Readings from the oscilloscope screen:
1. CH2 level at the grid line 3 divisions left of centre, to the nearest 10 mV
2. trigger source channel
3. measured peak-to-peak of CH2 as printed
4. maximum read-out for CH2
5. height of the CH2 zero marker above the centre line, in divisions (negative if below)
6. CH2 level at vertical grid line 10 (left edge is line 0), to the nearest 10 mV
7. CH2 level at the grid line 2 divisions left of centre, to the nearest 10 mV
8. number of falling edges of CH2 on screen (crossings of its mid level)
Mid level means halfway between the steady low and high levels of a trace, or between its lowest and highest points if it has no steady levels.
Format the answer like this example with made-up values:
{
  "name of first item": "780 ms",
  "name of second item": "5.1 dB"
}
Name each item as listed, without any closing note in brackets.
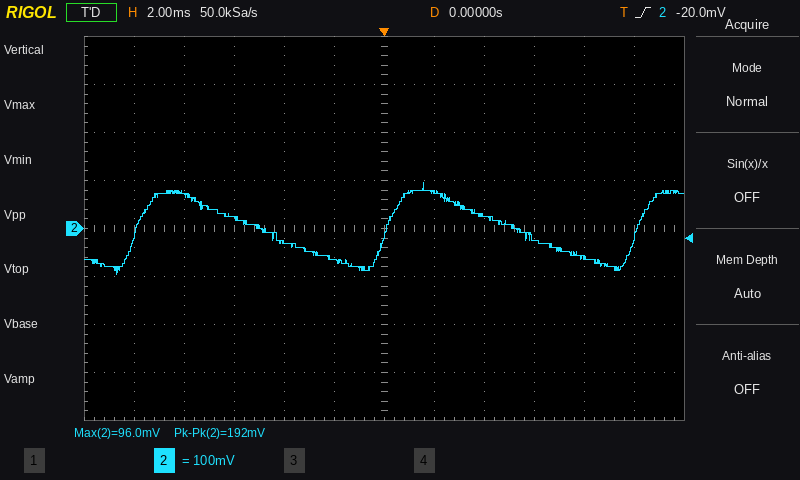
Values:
{
  "CH2 level at the grid line 3 divisions left of centre, to the nearest 10 mV": "20 mV",
  "trigger source channel": "CH2",
  "measured peak-to-peak of CH2 as printed": "192 mV",
  "maximum read-out for CH2": "96.0 mV",
  "height of the CH2 zero marker above the centre line, in divisions": "0.0 div",
  "CH2 level at vertical grid line 10 (left edge is line 0), to the nearest 10 mV": "-60 mV",
  "CH2 level at the grid line 2 divisions left of centre, to the nearest 10 mV": "-30 mV",
  "number of falling edges of CH2 on screen": "2"
}
